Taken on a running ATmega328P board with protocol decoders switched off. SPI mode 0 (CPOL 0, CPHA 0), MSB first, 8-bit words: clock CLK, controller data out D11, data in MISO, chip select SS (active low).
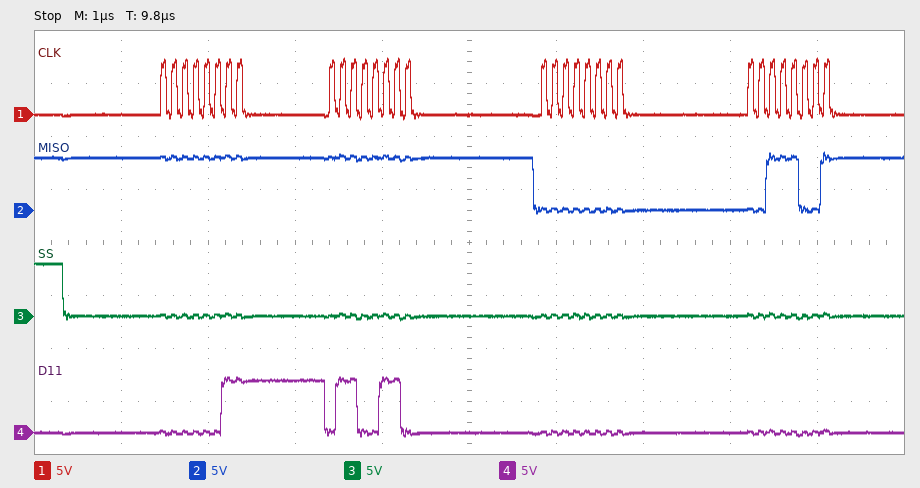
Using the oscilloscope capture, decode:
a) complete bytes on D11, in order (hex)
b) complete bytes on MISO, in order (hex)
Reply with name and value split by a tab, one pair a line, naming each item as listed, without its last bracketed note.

complete bytes on D11, in order	0x03 0x66 0x00 0x00
complete bytes on MISO, in order	0xFF 0xFF 0x00 0x39
